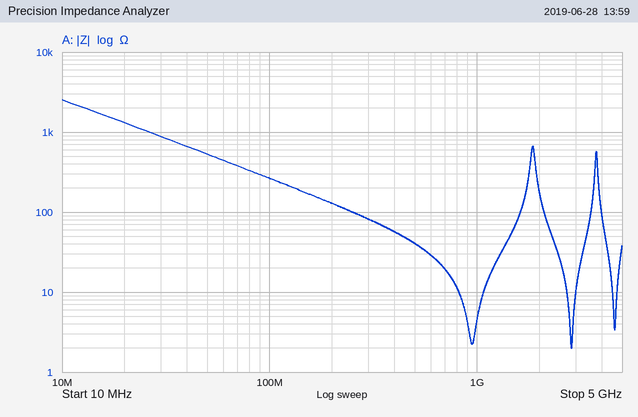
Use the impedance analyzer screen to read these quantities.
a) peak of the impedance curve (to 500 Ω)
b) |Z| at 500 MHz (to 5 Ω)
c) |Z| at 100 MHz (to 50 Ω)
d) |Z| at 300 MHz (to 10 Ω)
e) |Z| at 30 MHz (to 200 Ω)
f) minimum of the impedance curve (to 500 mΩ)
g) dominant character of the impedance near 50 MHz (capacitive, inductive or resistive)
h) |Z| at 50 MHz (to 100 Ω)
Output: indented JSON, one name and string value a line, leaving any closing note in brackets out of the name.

{
  "peak of the impedance curve": "2.5 kΩ",
  "|Z| at 500 MHz": "40 Ω",
  "|Z| at 100 MHz": "250 Ω",
  "|Z| at 300 MHz": "80 Ω",
  "|Z| at 30 MHz": "800 Ω",
  "minimum of the impedance curve": "2.0 Ω",
  "dominant character of the impedance near 50 MHz": "capacitive",
  "|Z| at 50 MHz": "500 Ω"
}
